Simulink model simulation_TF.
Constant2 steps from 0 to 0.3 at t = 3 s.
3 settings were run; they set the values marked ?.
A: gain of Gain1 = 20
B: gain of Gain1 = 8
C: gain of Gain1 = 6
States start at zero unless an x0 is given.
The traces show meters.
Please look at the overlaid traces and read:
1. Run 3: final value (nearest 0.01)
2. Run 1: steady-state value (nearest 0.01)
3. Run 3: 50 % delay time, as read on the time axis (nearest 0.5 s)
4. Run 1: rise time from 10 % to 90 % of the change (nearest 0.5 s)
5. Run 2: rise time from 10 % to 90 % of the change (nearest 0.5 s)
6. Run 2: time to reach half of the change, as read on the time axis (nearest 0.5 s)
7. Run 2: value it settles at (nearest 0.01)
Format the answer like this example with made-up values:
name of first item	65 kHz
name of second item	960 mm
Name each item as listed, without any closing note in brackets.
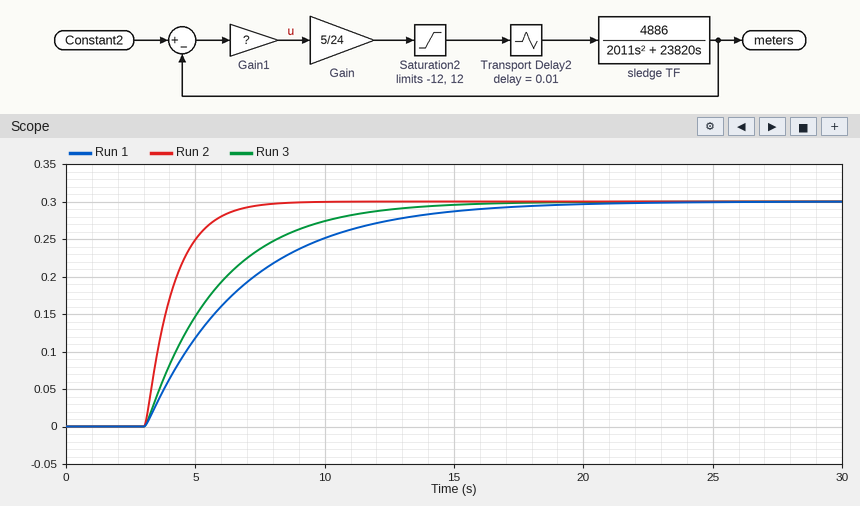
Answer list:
Run 3: final value	0.30
Run 1: steady-state value	0.30
Run 3: 50 % delay time, as read on the time axis	5.0 s
Run 1: rise time from 10 % to 90 % of the change	8.5 s
Run 2: rise time from 10 % to 90 % of the change	2.5 s
Run 2: time to reach half of the change, as read on the time axis	4.0 s
Run 2: value it settles at	0.30
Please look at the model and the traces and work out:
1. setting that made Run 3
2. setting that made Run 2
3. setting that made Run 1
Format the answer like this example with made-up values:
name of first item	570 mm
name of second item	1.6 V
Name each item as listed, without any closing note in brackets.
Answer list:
setting that made Run 3	B
setting that made Run 2	A
setting that made Run 1	C
